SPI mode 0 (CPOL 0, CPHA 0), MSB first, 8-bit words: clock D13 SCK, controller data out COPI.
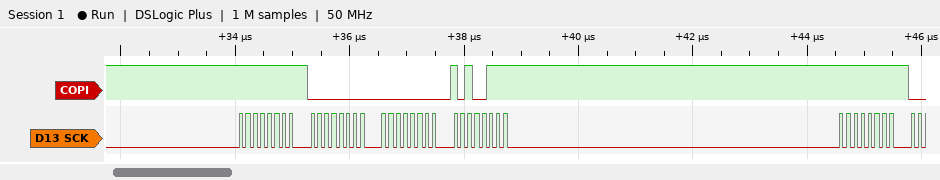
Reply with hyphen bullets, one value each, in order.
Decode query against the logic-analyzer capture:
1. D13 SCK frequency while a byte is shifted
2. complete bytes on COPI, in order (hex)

- 8 MHz
- FF 00 00 A7 FF
